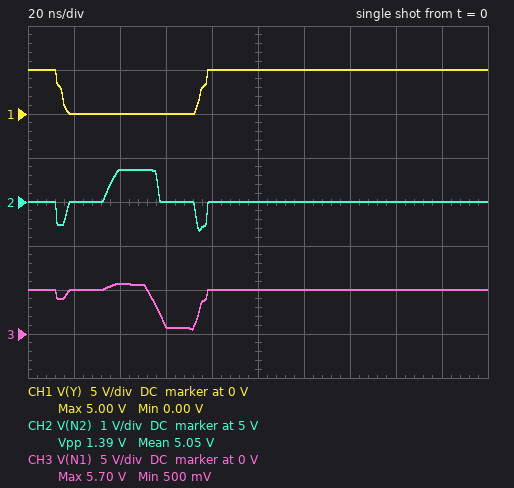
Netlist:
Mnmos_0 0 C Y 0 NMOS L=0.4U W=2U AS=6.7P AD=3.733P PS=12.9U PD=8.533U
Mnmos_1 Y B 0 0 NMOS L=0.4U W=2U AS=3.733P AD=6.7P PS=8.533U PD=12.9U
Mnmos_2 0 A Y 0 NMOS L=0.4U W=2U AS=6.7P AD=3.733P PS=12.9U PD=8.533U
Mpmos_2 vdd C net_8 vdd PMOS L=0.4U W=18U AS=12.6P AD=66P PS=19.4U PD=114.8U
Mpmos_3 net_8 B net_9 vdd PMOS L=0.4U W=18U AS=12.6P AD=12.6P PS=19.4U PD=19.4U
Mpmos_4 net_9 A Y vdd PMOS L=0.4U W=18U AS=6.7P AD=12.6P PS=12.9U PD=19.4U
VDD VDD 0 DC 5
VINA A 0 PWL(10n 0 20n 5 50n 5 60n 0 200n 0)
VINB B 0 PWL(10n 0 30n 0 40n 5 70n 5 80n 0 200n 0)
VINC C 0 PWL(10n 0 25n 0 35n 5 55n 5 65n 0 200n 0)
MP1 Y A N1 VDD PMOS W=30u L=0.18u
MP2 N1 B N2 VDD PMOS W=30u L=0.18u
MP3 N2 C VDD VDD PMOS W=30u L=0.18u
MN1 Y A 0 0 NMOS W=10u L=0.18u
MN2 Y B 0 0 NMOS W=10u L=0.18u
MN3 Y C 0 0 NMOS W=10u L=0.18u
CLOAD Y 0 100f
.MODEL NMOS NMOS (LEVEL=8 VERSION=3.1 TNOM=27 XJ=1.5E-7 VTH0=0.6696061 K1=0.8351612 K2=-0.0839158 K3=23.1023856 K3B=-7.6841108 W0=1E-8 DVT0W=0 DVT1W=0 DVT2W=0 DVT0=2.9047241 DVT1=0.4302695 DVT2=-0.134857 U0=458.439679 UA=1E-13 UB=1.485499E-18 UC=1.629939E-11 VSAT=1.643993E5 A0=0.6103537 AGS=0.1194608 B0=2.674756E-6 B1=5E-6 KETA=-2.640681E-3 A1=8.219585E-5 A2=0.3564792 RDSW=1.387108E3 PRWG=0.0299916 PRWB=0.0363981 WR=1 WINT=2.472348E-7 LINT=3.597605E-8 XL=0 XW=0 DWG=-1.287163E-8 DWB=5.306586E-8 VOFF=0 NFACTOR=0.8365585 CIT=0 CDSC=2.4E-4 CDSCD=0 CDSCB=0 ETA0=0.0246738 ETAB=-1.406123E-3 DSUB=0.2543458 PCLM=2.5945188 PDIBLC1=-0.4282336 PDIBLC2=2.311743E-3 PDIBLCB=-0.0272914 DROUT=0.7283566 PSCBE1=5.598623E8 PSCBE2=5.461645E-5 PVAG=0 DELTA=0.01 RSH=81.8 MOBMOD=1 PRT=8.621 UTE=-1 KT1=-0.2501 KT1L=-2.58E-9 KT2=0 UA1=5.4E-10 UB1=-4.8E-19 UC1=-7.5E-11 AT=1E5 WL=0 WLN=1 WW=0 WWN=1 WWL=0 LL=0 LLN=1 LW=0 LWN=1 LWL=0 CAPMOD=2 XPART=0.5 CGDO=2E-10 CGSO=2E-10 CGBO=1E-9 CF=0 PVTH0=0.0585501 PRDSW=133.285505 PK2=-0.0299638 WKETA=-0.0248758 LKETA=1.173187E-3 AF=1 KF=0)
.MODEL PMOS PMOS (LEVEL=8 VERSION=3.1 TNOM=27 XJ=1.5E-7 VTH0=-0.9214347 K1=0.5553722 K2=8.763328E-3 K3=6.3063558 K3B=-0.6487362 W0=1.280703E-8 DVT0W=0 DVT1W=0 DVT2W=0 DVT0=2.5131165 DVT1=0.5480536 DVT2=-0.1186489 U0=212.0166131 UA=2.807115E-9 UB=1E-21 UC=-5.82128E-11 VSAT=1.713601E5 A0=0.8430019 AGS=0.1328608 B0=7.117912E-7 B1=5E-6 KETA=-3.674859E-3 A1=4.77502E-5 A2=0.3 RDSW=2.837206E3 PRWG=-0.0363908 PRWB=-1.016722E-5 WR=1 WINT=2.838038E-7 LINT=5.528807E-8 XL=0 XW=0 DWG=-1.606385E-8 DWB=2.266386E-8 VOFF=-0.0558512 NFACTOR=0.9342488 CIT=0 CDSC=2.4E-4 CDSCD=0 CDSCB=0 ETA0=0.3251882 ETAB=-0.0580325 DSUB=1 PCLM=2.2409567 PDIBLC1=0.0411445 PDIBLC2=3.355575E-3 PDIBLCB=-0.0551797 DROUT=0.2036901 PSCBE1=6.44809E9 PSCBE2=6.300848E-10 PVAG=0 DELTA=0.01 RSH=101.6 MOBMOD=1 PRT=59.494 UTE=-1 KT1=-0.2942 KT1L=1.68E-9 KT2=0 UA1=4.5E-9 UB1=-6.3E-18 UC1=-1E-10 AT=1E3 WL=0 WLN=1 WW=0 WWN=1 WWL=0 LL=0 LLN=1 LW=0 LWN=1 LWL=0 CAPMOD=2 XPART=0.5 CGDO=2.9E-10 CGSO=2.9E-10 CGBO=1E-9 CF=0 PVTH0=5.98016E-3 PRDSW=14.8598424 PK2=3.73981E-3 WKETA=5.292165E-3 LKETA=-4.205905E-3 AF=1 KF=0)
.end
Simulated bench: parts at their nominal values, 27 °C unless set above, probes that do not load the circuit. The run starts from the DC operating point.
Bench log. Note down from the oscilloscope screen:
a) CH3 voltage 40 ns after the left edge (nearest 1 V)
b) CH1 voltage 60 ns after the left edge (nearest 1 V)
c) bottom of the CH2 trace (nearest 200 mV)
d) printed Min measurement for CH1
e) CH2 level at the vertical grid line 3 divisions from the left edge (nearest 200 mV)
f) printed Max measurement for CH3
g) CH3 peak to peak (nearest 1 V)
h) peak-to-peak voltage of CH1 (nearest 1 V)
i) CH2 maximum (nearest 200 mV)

6 V
0 V
4.4 V
0.00 V
5.0 V
5.70 V
5 V
5 V
5.8 V
